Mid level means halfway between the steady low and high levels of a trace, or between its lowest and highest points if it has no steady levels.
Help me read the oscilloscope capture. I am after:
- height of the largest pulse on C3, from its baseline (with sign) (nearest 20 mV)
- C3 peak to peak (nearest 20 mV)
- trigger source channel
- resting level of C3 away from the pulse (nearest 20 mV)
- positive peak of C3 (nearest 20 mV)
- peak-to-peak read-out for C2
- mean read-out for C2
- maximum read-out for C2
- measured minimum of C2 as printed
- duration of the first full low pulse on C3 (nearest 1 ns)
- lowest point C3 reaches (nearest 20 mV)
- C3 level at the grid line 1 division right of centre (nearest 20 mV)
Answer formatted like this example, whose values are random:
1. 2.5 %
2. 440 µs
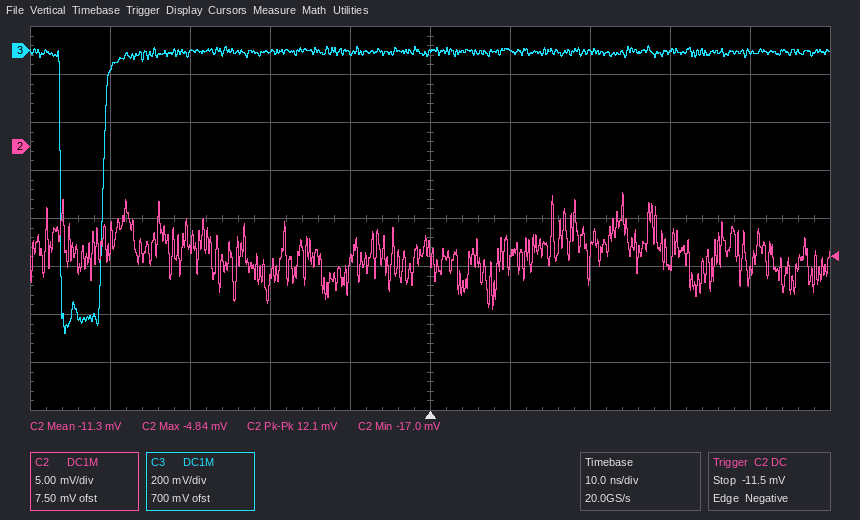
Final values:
1. -1.18 V
2. 1.20 V
3. C2
4. 0 mV
5. 20 mV
6. 12.1 mV
7. -11.3 mV
8. -4.84 mV
9. -17.0 mV
10. 5 ns
11. -1.18 V
12. 0 mV
